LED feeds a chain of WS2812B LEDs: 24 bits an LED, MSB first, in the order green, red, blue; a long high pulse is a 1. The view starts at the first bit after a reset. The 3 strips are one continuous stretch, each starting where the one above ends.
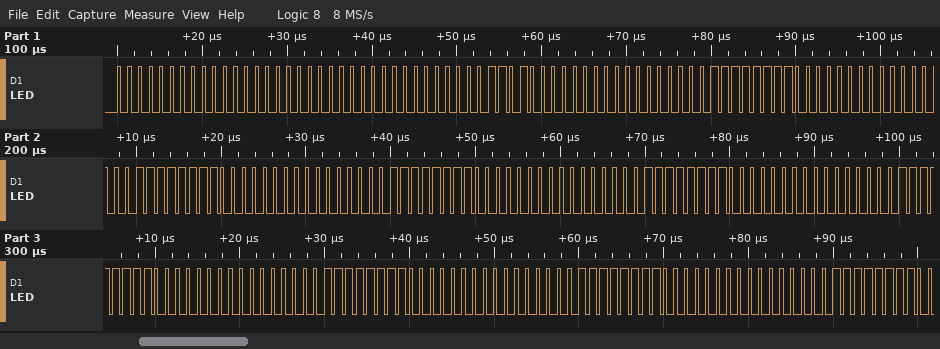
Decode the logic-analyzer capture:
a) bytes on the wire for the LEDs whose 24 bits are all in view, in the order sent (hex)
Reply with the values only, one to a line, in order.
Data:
00 00 00 00 1A 00 00 FF 00 00 FF 00 00 FF 00 00 FF 00 00 FF 00 00 FF 00 00 FF 00
